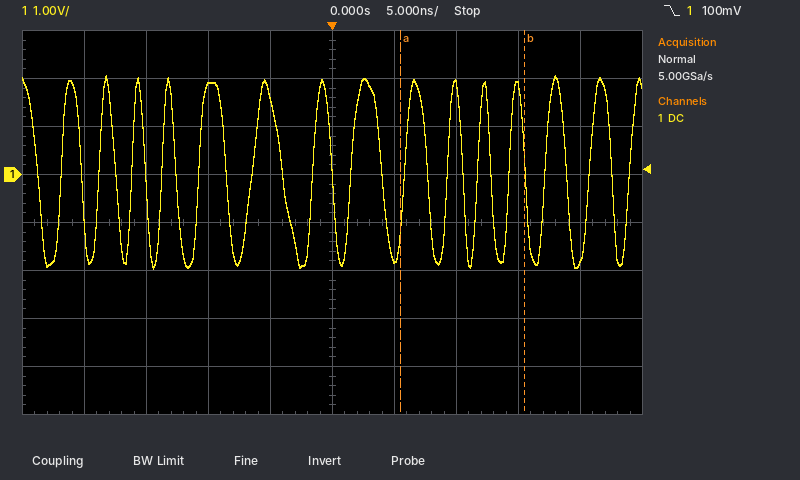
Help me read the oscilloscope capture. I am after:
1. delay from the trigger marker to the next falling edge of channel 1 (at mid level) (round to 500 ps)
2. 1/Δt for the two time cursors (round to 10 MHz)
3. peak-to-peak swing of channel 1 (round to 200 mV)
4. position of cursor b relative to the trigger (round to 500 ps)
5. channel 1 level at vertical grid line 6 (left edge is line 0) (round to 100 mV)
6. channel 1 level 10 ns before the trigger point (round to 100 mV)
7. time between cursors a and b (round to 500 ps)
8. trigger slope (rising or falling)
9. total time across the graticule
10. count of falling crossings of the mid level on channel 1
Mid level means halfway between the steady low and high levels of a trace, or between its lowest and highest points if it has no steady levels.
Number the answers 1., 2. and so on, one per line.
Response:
1. 4.0 ns
2. 100 MHz
3. 4.0 V
4. +15.5 ns
5. -1.7 V
6. 1.8 V
7. 10.0 ns
8. falling
9. 50 ns
10. 15
